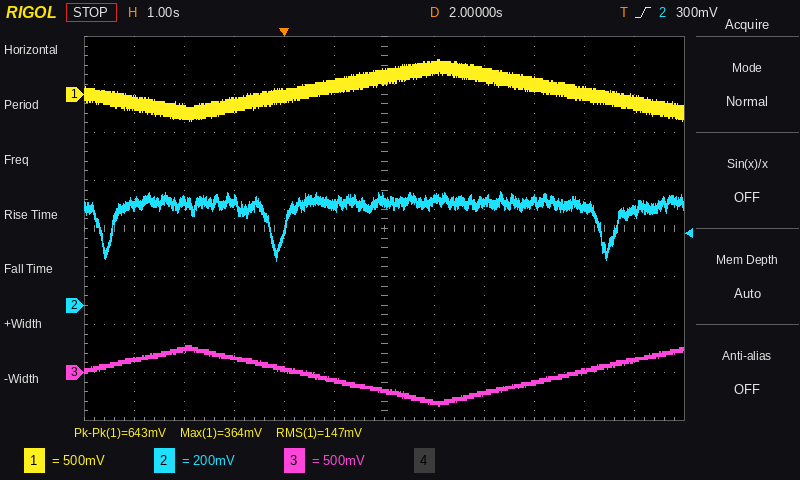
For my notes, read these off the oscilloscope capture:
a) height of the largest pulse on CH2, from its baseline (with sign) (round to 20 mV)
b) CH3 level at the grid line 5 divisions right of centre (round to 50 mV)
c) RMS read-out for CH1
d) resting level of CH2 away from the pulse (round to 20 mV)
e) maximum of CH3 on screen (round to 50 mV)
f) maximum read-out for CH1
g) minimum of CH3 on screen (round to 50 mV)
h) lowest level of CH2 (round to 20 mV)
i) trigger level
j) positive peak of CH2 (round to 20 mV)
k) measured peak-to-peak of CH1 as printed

-240 mV
150 mV
147 mV
420 mV
300 mV
364 mV
-350 mV
180 mV
300 mV
480 mV
643 mV
